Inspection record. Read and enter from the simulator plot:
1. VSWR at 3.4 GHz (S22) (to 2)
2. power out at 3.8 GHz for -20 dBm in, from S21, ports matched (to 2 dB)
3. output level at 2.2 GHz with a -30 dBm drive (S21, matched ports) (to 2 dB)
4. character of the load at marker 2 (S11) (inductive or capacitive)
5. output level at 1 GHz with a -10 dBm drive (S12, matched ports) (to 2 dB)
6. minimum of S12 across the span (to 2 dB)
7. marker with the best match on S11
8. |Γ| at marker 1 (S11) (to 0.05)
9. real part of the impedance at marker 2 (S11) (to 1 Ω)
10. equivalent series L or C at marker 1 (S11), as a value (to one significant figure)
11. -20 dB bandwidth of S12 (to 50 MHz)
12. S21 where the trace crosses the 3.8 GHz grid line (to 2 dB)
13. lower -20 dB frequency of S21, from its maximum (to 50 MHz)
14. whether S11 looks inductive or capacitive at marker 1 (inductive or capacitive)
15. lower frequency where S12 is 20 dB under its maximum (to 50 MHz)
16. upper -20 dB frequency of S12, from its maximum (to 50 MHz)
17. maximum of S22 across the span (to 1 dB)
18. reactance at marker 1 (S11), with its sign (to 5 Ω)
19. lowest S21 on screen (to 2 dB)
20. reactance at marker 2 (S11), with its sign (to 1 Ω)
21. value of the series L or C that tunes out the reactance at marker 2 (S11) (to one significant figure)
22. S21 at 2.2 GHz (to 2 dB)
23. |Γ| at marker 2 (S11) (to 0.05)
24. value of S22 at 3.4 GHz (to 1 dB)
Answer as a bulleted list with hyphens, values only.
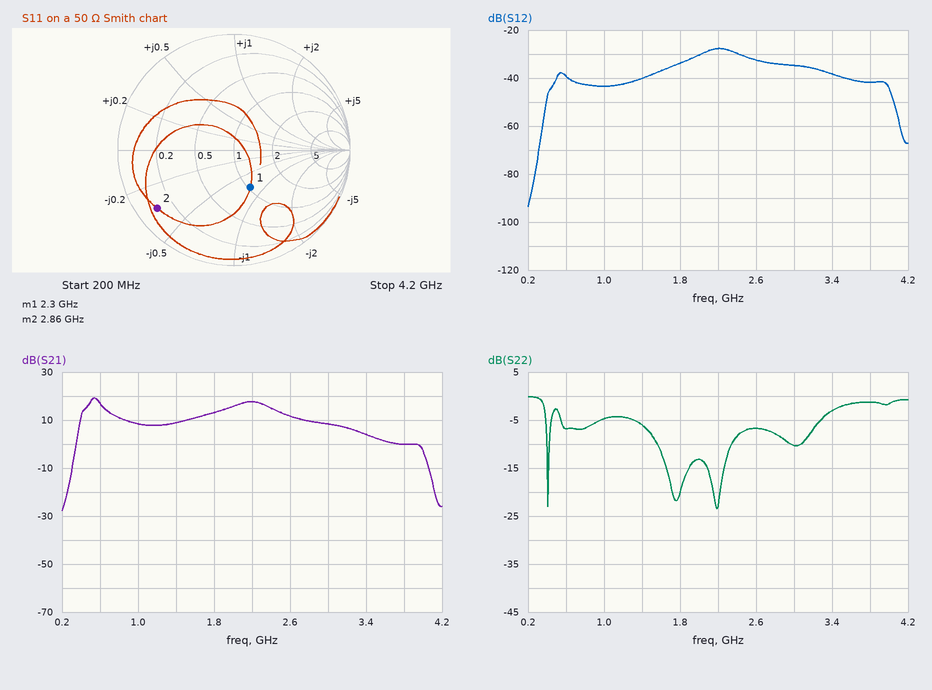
- 6
- -20 dBm
- -12 dBm
- capacitive
- -54 dBm
- -94 dB
- marker 1
- 0.35
- 5 Ω
- 2 pF
- 3.65 GHz
- 0 dB
- 350 MHz
- capacitive
- 400 MHz
- 4.05 GHz
- 0 dB
- -40 Ω
- -28 dB
- -17 Ω
- 900 pH
- 18 dB
- 0.85
- -3 dB
